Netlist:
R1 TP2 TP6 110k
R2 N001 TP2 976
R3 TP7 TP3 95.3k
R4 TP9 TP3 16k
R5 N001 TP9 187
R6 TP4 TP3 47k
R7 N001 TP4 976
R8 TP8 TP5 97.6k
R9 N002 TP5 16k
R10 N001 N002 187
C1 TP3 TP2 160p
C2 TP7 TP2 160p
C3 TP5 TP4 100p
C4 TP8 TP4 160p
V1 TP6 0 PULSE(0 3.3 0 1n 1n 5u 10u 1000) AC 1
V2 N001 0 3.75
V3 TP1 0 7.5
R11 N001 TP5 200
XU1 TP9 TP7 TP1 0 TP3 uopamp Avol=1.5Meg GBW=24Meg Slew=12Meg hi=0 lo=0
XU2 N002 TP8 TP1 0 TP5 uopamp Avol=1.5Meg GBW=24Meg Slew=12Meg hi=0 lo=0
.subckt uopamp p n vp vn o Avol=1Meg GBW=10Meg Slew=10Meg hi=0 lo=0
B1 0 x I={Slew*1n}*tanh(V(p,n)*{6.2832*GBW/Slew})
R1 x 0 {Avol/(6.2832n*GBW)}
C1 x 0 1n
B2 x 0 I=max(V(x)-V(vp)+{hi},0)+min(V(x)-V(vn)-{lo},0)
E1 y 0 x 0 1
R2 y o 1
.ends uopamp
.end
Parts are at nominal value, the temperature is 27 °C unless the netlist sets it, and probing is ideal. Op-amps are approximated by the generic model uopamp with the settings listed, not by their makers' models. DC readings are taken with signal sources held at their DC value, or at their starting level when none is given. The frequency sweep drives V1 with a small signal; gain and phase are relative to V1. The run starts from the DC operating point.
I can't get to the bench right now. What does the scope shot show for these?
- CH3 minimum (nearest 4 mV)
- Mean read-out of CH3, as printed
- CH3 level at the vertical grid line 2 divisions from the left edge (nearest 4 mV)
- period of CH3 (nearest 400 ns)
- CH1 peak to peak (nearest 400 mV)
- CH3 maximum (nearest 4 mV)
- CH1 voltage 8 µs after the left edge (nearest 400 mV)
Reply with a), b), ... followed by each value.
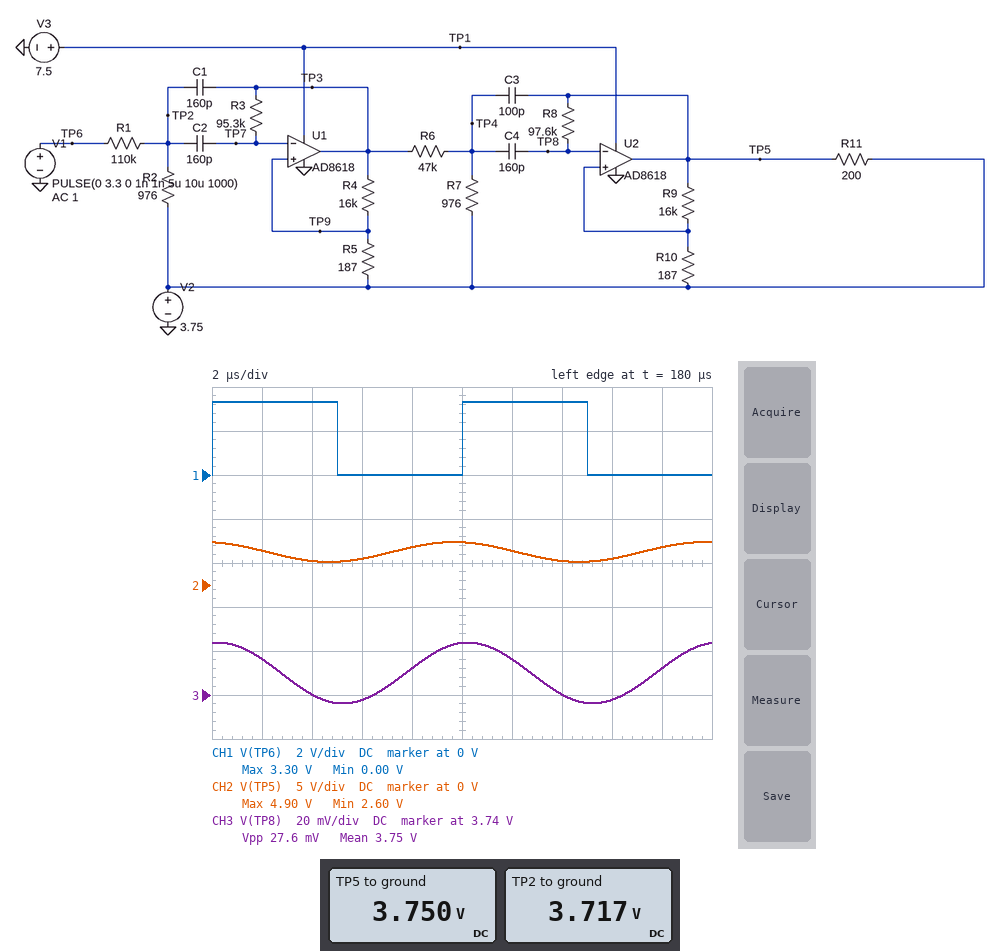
a) 3.736 V
b) 3.75 V
c) 3.740 V
d) 10.0 µs
e) 3.2 V
f) 3.764 V
g) 0 V
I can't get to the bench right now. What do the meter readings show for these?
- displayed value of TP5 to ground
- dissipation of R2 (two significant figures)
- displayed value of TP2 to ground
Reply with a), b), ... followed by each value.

a) 3.750 V
b) 1.1 µW
c) 3.717 V
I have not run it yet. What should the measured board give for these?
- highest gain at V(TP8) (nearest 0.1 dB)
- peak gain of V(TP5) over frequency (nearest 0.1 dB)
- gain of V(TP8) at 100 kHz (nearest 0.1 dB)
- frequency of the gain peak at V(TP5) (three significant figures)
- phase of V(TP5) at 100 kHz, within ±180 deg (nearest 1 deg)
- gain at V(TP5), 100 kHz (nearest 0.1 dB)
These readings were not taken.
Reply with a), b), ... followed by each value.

a) -38.4 dB
b) -0.5 dB
c) -43.7 dB
d) 125 kHz
e) 101 deg
f) -5.5 dB
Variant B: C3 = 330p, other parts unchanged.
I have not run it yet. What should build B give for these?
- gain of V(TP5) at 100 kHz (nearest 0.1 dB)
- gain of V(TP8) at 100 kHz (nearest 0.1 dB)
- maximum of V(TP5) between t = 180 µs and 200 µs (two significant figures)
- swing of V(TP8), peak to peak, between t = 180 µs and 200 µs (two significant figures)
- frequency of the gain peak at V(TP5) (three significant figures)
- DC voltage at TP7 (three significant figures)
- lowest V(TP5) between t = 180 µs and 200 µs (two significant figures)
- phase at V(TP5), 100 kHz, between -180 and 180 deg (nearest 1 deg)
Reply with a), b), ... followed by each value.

a) -14.1 dB
b) -52.3 dB
c) 4.2 V
d) 10 mV
e) 101 kHz
f) 3.75 V
g) 3.3 V
h) -62 deg
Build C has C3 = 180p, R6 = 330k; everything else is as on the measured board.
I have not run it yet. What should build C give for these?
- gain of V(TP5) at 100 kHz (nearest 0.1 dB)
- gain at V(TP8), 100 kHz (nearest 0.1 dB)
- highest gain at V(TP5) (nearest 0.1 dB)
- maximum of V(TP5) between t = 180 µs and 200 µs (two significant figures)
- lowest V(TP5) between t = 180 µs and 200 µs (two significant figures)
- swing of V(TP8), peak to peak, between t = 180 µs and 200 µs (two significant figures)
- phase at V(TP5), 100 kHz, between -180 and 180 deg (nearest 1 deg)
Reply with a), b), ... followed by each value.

a) -14.6 dB
b) -52.8 dB
c) -14.4 dB
d) 4.1 V
e) 3.4 V
f) 9.6 mV
g) -35 deg
